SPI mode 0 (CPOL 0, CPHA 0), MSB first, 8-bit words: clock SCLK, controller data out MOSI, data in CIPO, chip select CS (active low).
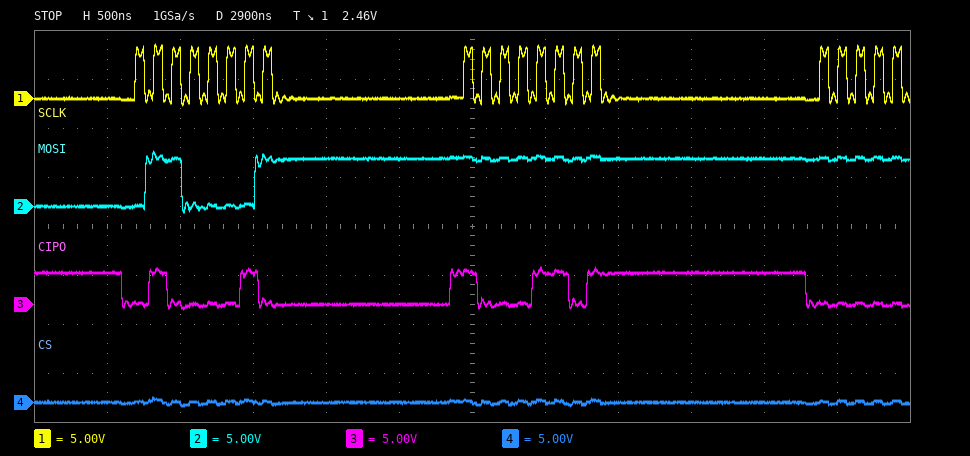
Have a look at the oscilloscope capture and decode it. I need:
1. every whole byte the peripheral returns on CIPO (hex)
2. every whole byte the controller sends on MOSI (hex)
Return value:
42 8D
61 FF
